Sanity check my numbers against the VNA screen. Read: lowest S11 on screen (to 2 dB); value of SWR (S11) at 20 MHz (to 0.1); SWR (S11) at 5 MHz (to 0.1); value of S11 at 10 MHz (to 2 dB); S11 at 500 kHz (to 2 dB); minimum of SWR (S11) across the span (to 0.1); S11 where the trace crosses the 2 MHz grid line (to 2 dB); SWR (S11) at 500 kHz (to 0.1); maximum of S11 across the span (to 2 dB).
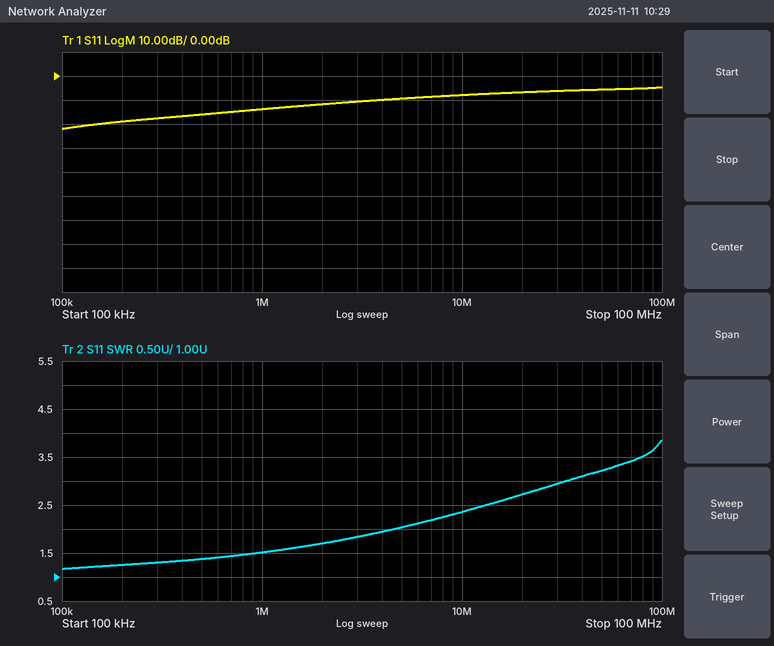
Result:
-22 dB
2.7
2.0
-8 dB
-16 dB
1.2
-12 dB
1.4
-4 dB
